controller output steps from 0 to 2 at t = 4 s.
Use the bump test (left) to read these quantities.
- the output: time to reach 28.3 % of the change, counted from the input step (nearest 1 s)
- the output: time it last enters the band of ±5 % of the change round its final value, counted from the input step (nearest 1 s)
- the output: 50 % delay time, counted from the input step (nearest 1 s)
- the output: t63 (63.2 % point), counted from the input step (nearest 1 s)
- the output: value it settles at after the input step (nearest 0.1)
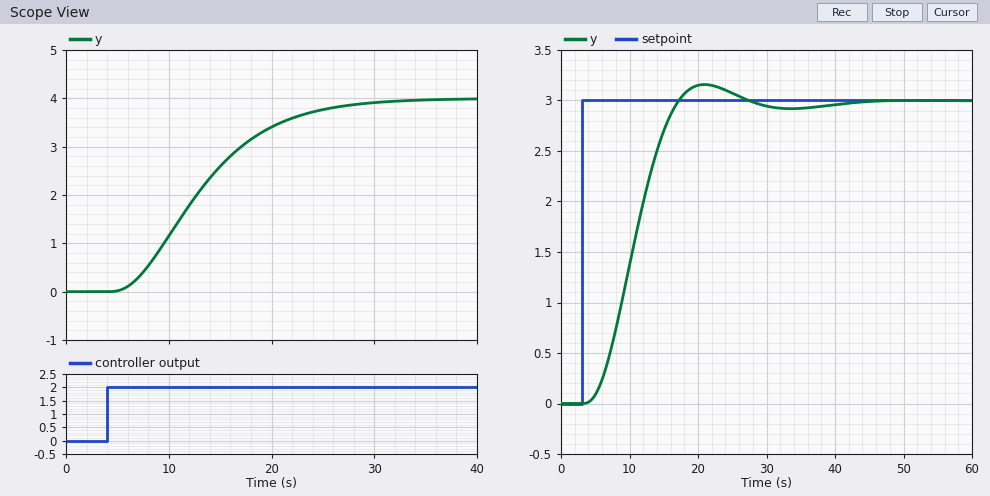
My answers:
6 s
22 s
9 s
11 s
4.0
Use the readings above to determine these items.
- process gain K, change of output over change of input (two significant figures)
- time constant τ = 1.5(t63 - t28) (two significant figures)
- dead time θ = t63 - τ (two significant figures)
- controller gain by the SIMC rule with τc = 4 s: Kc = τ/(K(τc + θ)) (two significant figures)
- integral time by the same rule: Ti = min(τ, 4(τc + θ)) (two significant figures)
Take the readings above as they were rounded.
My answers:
2.0
7.5 s
3.5 s
0.50
7.5 s
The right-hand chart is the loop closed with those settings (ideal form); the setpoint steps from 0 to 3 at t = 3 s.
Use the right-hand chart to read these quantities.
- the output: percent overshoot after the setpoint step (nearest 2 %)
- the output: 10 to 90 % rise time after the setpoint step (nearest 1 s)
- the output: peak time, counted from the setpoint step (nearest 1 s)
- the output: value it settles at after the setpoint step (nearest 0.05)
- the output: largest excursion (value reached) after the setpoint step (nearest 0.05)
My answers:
6 %
9 s
18 s
3.00
3.15
